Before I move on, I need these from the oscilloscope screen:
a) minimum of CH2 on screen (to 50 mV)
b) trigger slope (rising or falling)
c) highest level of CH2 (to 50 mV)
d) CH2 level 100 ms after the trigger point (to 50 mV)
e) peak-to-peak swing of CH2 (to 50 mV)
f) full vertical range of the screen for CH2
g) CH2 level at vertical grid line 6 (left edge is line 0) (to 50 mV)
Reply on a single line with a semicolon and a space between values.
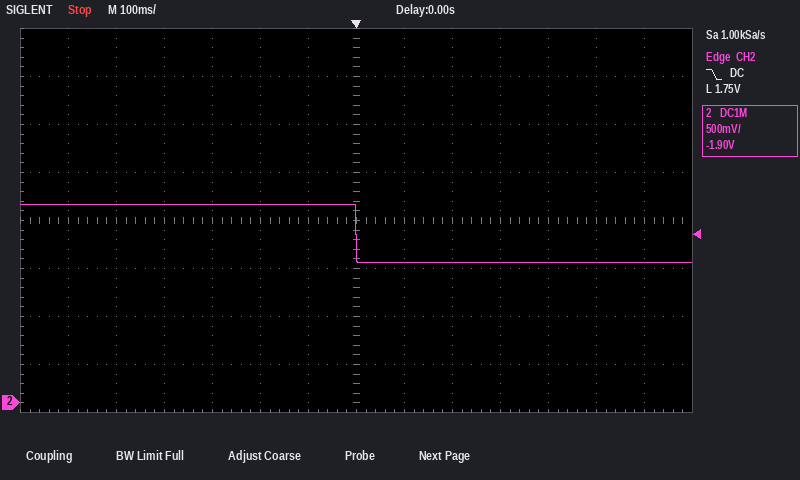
1.45 V; falling; 2.05 V; 1.45 V; 600 mV; 4 V; 2.05 V
